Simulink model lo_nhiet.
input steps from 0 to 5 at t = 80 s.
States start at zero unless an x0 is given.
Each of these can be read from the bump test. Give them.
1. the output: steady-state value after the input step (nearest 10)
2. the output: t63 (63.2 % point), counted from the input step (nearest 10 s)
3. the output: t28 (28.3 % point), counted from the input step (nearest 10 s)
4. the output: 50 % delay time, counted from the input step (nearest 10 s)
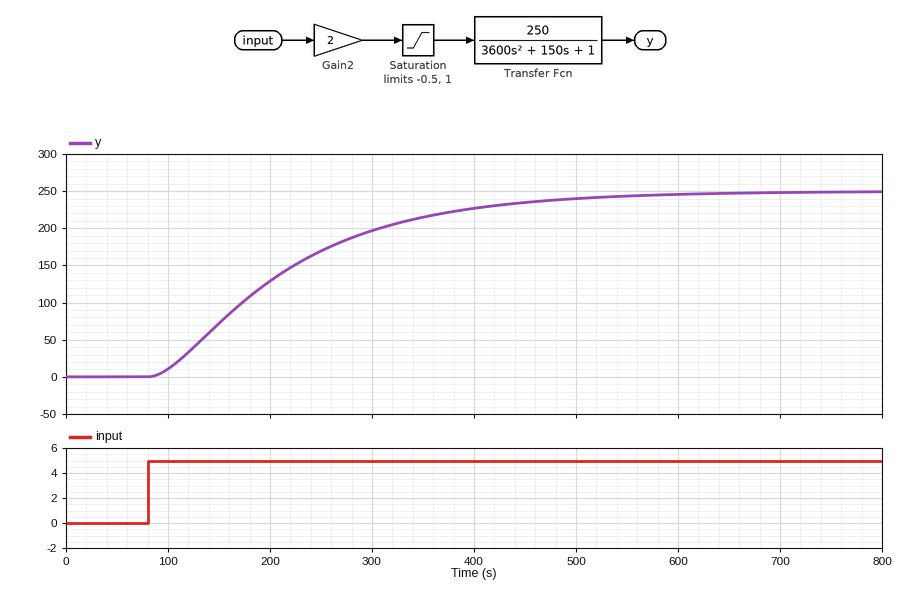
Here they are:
250
150 s
70 s
120 s
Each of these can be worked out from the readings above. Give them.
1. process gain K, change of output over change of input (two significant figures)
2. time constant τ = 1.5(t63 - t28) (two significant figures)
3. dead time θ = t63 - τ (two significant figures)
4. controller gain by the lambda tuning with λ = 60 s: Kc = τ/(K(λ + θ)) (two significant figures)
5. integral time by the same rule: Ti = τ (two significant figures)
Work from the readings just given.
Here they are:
50
120 s
30 s
0.027
120 s
